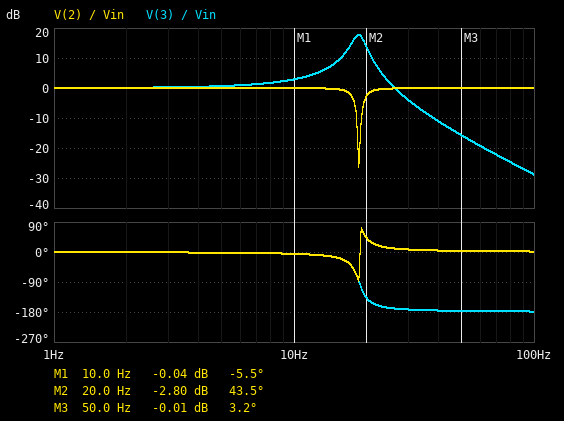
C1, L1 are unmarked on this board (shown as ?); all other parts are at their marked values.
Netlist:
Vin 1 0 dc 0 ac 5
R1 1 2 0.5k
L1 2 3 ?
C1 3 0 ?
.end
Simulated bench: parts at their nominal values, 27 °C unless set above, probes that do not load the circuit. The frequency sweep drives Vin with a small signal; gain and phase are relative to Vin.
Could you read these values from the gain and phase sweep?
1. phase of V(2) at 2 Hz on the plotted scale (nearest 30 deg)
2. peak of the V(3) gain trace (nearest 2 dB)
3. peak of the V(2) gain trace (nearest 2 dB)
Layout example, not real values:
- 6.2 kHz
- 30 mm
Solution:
- 0 deg
- 18 dB
- 0 dB
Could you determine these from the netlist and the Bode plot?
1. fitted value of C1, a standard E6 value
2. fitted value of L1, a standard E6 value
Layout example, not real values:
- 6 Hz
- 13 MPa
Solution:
- 2.2 µF
- 33 H
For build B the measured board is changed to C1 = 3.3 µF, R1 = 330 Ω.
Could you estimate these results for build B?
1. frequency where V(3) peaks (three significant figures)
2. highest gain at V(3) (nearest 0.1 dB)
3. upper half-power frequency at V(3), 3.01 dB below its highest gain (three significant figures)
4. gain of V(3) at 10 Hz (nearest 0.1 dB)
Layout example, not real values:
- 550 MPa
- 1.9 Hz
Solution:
- 15.2 Hz
- 19.6 dB
- 16.0 Hz
- 4.8 dB
